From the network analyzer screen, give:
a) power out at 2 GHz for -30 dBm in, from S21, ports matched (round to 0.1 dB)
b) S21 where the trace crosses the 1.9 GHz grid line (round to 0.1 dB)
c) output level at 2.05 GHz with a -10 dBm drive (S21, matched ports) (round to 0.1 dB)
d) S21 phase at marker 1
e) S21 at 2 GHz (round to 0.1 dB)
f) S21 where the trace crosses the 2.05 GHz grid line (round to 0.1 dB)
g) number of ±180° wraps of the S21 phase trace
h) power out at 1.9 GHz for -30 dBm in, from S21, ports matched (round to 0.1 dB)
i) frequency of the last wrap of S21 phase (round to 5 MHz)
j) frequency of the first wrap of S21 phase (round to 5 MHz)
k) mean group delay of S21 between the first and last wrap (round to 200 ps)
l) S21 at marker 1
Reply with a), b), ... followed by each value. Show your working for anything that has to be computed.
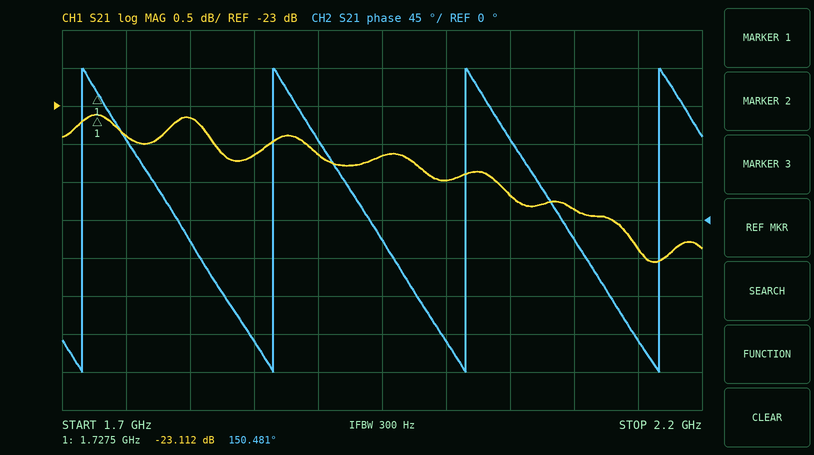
a) -30 dBm + (-24.0 dB) = -54.0 dBm
b) -23.6 dB
c) -10 dBm + (-24.2 dB) = -34.2 dBm
d) 150.481°
e) -24.0 dB
f) -24.2 dB
g) 4
h) -30 dBm + (-23.6 dB) = -53.6 dBm
i) 2.165 GHz
j) 1.715 GHz
k) 3 cycles / (2.165 GHz − 1.715 GHz) ≈ 6.67 ns, so 6.6 ns to the nearest 200 ps
l) -23.112 dB
